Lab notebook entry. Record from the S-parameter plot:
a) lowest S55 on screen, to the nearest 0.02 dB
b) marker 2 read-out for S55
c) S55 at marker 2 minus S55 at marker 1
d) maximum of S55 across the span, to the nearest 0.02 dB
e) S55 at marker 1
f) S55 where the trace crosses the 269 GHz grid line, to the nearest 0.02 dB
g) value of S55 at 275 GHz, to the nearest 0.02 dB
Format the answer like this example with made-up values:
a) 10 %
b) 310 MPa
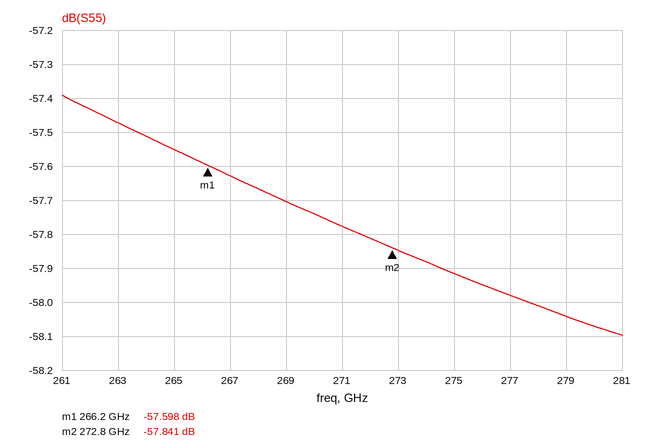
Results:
a) -58.10 dB
b) -57.841 dB
c) -0.243 dB
d) -57.40 dB
e) -57.598 dB
f) -57.70 dB
g) -57.92 dB
